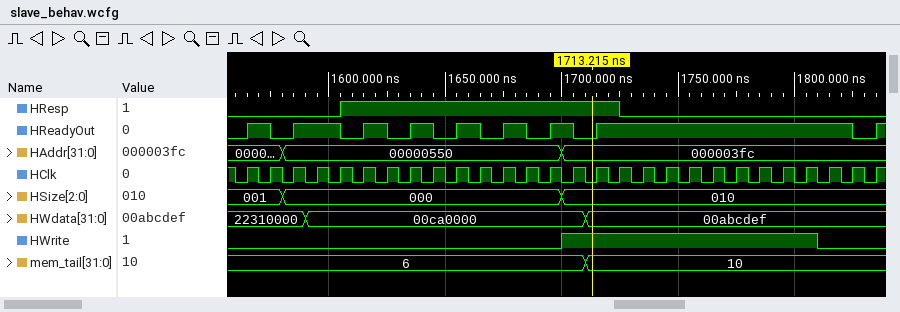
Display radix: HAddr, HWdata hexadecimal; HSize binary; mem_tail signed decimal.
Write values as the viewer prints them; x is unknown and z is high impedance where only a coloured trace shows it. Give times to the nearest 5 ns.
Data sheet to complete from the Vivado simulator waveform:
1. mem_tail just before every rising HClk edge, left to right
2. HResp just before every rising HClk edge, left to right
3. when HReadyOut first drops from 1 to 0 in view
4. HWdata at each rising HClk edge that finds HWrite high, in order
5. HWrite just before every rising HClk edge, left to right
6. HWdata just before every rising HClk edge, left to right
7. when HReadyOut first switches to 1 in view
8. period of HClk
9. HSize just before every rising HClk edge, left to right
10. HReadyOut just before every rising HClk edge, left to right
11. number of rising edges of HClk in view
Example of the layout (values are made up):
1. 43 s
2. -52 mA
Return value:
1. 6, 6, 6, 6, 6, 6, 6, 6, 6, 6, 6, 6, 6, 6, 6, 10, 10, 10, 10, 10, 10, 10, 10, 10, 10, 10, 10, 10
2. 0 0 0 0 0 1 1 1 1 1 1 1 1 1 1 1 1 0 0 0 0 0 0 0 0 0 0 0
3. 1575 ns
4. 00ca0000, 00abcdef, 00abcdef, 00abcdef, 00abcdef, 00abcdef, 00abcdef, 00abcdef, 00abcdef, 00abcdef, 00abcdef
5. 0 0 0 0 0 0 0 0 0 0 0 0 0 0 1 1 1 1 1 1 1 1 1 1 1 0 0 0
6. 22310000, 22310000, 22310000, 00ca0000, 00ca0000, 00ca0000, 00ca0000, 00ca0000, 00ca0000, 00ca0000, 00ca0000, 00ca0000, 00ca0000, 00ca0000, 00ca0000, 00abcdef, 00abcdef, 00abcdef, 00abcdef, 00abcdef, 00abcdef, 00abcdef, 00abcdef, 00abcdef, 00abcdef, 00abcdef, 00abcdef, 00abcdef
7. 1565 ns
8. 10 ns
9. 001, 001, 000, 000, 000, 000, 000, 000, 000, 000, 000, 000, 000, 000, 010, 010, 010, 010, 010, 010, 010, 010, 010, 010, 010, 010, 010, 010
10. 0 1 0 1 1 0 1 0 1 0 1 0 1 0 1 0 1 1 1 1 1 1 1 1 1 1 1 0
11. 28
